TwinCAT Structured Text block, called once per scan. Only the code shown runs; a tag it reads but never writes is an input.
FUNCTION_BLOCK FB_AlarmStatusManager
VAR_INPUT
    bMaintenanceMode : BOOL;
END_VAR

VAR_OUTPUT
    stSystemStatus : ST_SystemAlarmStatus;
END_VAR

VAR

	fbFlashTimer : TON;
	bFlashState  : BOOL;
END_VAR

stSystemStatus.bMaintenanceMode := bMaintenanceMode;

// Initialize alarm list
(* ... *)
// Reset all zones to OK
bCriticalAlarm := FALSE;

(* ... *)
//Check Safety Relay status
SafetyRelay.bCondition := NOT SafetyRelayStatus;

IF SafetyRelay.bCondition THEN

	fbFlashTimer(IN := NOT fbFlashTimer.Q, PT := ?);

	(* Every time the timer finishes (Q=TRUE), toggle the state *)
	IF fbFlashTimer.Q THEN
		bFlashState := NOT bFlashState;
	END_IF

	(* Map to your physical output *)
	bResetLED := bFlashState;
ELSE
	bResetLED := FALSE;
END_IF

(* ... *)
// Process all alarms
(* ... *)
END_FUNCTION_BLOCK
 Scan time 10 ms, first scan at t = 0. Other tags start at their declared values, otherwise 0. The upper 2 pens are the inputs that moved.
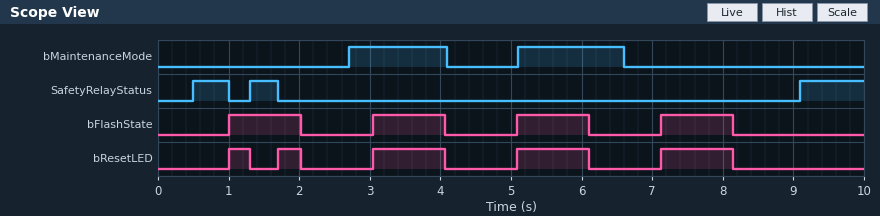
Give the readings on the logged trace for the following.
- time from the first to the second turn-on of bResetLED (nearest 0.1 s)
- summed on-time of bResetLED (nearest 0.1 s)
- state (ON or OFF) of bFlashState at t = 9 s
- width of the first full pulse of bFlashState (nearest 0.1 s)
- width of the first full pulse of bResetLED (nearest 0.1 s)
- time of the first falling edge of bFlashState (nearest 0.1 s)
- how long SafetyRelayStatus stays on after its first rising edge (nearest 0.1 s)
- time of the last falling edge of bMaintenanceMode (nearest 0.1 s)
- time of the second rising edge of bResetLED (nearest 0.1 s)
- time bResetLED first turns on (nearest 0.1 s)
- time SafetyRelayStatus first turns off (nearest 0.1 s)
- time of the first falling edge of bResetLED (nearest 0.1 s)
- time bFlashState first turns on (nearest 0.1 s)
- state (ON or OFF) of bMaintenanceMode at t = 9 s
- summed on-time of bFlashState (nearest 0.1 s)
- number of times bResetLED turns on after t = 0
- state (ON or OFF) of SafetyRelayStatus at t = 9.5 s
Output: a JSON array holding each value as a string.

["0.7 s", "3.7 s", "OFF", "1.0 s", "0.3 s", "2.0 s", "0.5 s", "6.6 s", "1.7 s", "1.0 s", "1.0 s", "1.3 s", "1.0 s", "OFF", "4.1 s", "5", "ON"]
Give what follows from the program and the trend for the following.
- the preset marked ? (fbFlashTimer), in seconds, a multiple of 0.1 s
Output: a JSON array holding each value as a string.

["1.0 s"]
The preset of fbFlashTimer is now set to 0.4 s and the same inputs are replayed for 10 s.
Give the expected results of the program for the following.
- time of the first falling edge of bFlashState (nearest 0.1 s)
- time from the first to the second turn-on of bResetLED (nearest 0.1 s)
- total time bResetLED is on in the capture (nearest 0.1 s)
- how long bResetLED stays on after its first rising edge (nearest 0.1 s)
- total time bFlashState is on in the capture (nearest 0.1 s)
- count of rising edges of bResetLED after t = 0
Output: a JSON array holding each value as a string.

["1.0 s", "1.3 s", "3.9 s", "0.1 s", "4.4 s", "10"]
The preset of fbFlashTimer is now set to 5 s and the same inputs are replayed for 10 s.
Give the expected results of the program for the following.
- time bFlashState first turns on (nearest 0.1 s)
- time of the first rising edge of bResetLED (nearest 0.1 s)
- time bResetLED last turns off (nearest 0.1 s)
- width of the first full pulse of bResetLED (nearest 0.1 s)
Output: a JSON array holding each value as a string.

["5.0 s", "5.0 s", "9.1 s", "4.1 s"]
